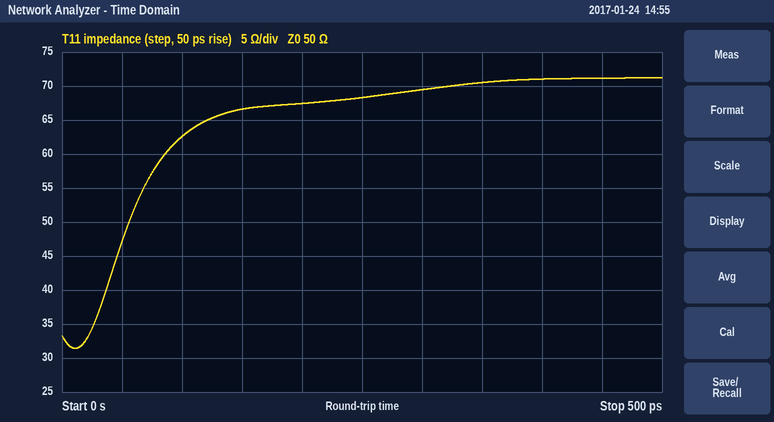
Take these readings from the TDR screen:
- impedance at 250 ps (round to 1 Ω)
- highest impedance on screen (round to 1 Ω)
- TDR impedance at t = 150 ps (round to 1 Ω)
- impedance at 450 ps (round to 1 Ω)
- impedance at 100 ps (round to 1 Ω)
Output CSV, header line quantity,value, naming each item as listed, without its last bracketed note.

quantity,value
impedance at 250 ps,68 Ω
highest impedance on screen,71 Ω
TDR impedance at t = 150 ps,67 Ω
impedance at 450 ps,71 Ω
impedance at 100 ps,63 Ω
